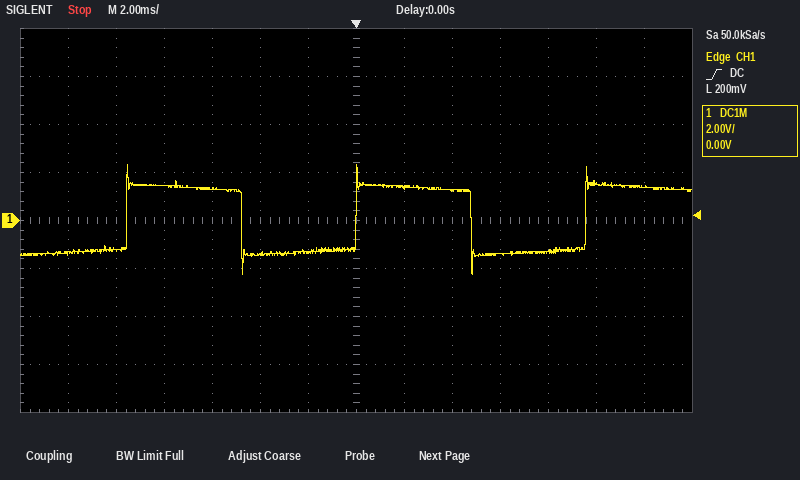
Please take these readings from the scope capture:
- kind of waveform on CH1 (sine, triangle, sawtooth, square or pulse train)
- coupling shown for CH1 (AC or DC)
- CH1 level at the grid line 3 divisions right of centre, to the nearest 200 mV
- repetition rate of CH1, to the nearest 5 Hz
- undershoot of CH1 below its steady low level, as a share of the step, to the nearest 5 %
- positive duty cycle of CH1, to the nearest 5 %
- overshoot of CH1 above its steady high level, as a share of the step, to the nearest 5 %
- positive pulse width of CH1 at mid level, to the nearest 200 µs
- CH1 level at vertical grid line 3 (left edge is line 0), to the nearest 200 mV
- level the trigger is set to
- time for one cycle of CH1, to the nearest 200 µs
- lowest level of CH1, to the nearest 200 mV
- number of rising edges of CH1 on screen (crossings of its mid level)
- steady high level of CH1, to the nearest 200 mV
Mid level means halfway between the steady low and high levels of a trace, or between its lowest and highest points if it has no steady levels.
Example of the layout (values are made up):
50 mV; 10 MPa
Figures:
square; DC; -1.4 V; 105 Hz; 35 %; 50 %; 35 %; 4.8 ms; 1.4 V; 200 mV; 9.6 ms; -2.2 V; 3; 1.4 V
